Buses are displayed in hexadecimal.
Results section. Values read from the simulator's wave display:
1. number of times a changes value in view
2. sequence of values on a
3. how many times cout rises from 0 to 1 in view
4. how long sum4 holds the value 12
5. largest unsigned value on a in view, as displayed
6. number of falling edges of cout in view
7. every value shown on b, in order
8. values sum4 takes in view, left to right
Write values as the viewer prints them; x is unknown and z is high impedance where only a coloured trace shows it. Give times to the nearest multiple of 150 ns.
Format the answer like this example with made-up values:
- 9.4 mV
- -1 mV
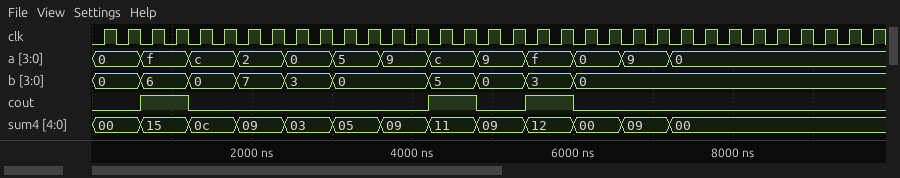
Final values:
- 12
- 0, f, c, 2, 0, 5, 9, c, 9, f, 0, 9, 0
- 3
- 600 ns
- f
- 3
- 0, 6, 0, 7, 3, 0, 5, 0, 3, 0
- 00, 15, 0c, 09, 03, 05, 09, 11, 09, 12, 00, 09, 00
